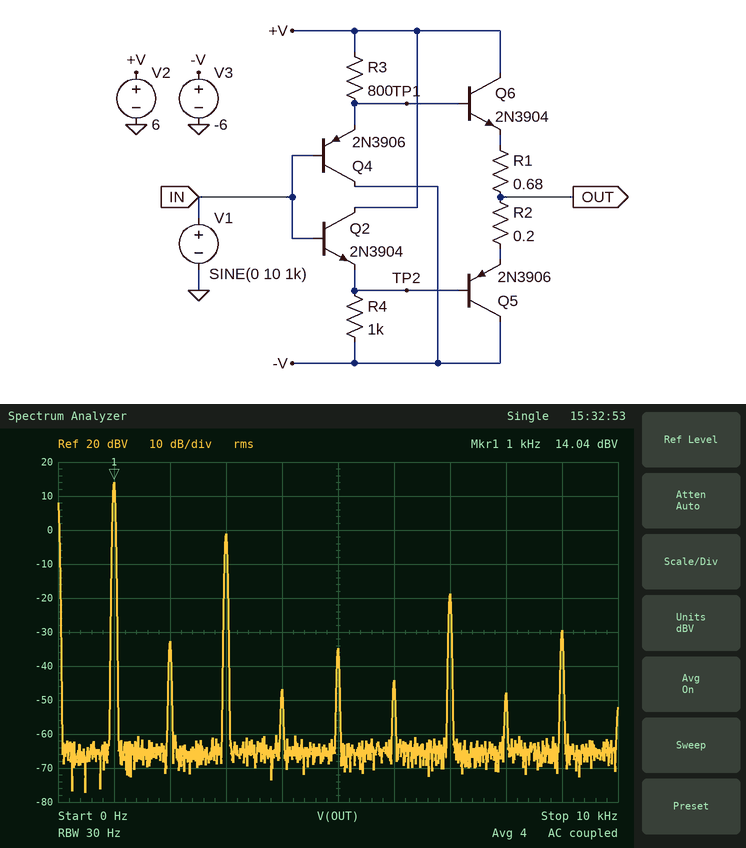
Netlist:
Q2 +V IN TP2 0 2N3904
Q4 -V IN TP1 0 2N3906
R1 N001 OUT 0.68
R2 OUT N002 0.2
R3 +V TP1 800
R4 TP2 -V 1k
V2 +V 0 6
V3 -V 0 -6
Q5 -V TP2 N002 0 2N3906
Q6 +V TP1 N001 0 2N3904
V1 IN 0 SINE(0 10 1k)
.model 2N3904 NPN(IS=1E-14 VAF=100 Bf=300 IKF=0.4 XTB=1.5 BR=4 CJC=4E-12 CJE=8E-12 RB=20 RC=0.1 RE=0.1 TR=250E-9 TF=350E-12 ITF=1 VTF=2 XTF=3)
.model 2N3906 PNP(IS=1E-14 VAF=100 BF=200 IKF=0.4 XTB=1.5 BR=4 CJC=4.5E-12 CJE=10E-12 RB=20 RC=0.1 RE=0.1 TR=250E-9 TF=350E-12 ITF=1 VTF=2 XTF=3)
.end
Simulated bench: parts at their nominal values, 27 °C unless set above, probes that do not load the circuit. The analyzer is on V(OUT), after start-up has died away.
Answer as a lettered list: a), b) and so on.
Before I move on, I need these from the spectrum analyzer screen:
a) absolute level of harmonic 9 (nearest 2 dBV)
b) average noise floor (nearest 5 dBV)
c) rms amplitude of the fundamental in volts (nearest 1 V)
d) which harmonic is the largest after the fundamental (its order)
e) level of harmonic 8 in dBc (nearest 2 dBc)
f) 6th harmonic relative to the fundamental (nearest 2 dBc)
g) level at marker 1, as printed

a) -30 dBV
b) -65 dBV
c) 5 V
d) 3
e) -62 dBc
f) -58 dBc
g) 14.04 dBV
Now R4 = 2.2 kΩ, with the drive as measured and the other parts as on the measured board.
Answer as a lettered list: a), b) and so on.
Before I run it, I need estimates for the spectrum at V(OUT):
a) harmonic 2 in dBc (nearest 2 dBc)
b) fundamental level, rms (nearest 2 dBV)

a) -48 dBc
b) 14 dBV
